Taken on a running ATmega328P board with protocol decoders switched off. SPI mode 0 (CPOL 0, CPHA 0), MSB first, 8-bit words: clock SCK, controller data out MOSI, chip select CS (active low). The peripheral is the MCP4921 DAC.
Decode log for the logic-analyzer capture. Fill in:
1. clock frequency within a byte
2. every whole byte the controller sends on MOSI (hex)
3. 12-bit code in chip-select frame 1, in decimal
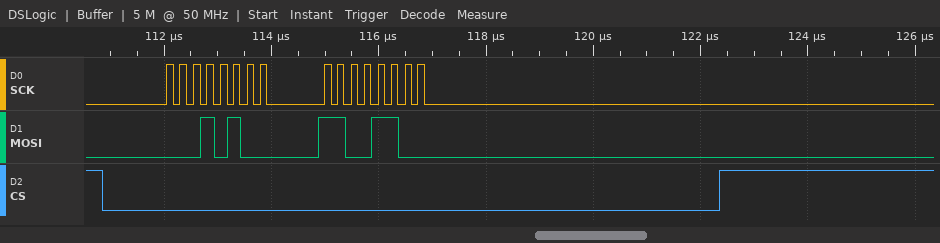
4 MHz
0x14 0xCC
1228
